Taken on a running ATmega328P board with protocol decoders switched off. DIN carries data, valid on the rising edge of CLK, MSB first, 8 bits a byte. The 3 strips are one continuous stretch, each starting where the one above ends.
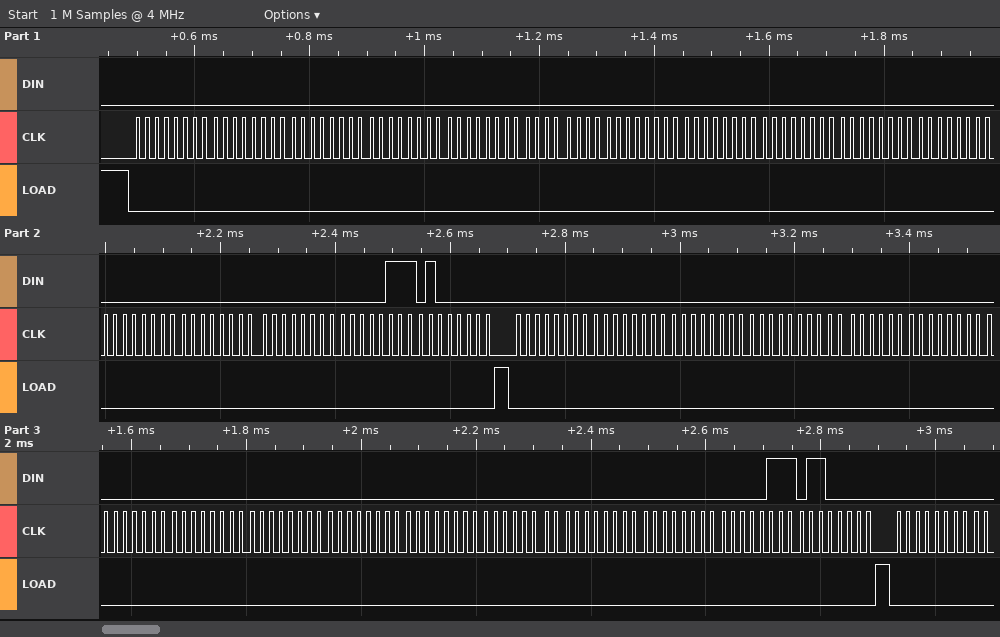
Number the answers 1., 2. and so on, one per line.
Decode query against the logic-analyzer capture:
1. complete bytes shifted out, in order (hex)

1. 00 00 00 00 00 00 00 00 00 00 00 00 00 00 07 40 00 00 00 00 00 00 00 00 00 00 00 00 00 00 07 60 00
